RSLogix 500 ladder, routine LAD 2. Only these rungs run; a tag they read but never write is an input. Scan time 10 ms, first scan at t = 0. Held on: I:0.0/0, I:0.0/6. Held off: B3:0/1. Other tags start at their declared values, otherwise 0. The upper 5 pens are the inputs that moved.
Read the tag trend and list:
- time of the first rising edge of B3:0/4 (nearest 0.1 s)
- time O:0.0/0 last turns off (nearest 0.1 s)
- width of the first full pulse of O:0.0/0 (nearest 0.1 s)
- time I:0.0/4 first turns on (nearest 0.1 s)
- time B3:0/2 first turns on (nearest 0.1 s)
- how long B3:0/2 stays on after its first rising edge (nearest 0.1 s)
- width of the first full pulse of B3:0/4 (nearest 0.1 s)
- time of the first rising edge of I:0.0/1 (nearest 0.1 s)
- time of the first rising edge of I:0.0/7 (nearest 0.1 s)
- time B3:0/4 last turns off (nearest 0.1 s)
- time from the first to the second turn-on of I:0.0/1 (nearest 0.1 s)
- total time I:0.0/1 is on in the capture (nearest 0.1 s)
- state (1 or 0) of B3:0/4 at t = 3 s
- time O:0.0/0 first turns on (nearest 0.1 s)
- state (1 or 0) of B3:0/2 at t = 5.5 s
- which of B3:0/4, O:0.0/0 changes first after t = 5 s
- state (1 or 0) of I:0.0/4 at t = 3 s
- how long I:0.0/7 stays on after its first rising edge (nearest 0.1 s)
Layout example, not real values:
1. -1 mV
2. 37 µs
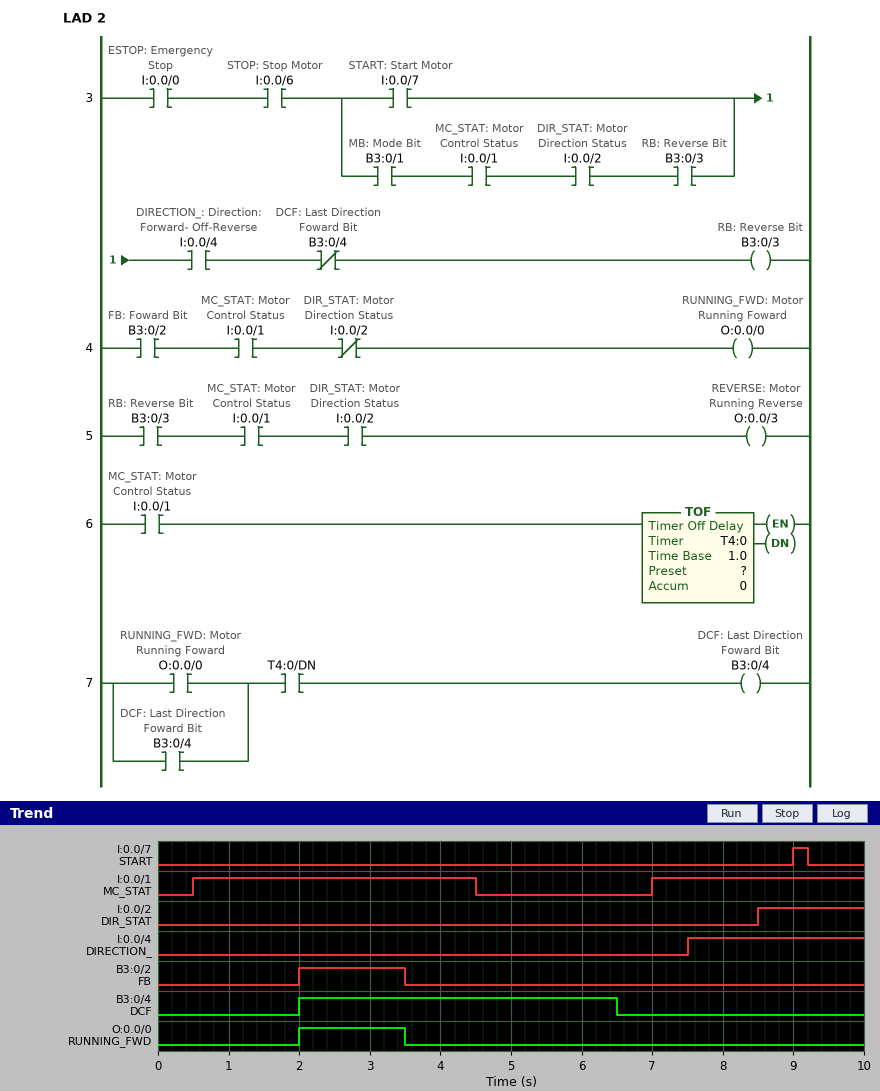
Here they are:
1. 2.0 s
2. 3.5 s
3. 1.5 s
4. 7.5 s
5. 2.0 s
6. 1.5 s
7. 4.5 s
8. 0.5 s
9. 9.0 s
10. 6.5 s
11. 6.5 s
12. 7.0 s
13. 1
14. 2.0 s
15. 0
16. B3:0/4
17. 0
18. 0.2 s
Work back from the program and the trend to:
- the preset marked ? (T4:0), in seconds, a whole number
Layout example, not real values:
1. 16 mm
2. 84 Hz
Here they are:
1. 2 s
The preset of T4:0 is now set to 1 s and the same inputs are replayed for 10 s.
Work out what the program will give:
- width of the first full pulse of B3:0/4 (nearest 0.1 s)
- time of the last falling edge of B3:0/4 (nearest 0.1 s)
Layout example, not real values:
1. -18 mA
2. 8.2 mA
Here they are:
1. 3.5 s
2. 5.5 s
